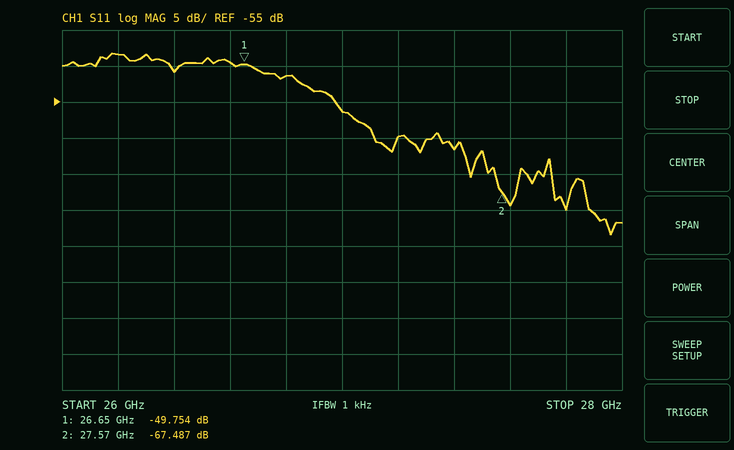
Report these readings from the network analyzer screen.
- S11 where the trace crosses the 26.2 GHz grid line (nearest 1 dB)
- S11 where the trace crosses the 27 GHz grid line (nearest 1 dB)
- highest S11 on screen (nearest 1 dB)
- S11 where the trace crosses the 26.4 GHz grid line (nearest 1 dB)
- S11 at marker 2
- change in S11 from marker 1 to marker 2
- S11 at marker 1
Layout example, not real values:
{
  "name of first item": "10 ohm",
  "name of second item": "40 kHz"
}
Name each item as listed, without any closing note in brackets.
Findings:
{
  "S11 where the trace crosses the 26.2 GHz grid line": "-48 dB",
  "S11 where the trace crosses the 27 GHz grid line": "-56 dB",
  "highest S11 on screen": "-48 dB",
  "S11 where the trace crosses the 26.4 GHz grid line": "-51 dB",
  "S11 at marker 2": "-67.487 dB",
  "change in S11 from marker 1 to marker 2": "-17.733 dB",
  "S11 at marker 1": "-49.754 dB"
}
